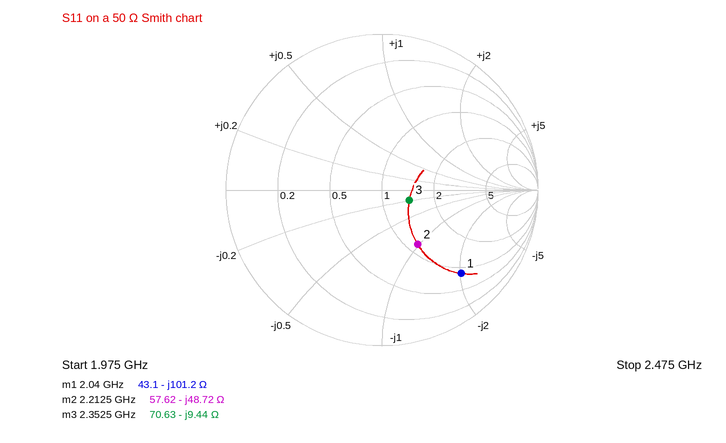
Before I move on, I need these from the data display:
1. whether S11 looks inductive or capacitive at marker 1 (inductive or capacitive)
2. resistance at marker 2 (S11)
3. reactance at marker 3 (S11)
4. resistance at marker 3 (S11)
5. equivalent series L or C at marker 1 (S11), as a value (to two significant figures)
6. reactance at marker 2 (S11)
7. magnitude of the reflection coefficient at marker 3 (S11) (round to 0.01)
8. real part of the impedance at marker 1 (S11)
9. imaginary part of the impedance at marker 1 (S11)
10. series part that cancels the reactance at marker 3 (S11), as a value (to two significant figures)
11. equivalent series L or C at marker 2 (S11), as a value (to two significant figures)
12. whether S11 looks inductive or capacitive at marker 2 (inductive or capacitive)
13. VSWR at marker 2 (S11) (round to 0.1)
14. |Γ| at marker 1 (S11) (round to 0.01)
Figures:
capacitive
57.62 Ω
-9.44 Ω
70.63 Ω
770 fF
-48.72 Ω
0.19
43.1 Ω
-101.2 Ω
640 pH
1.5 pF
capacitive
2.4
0.74
